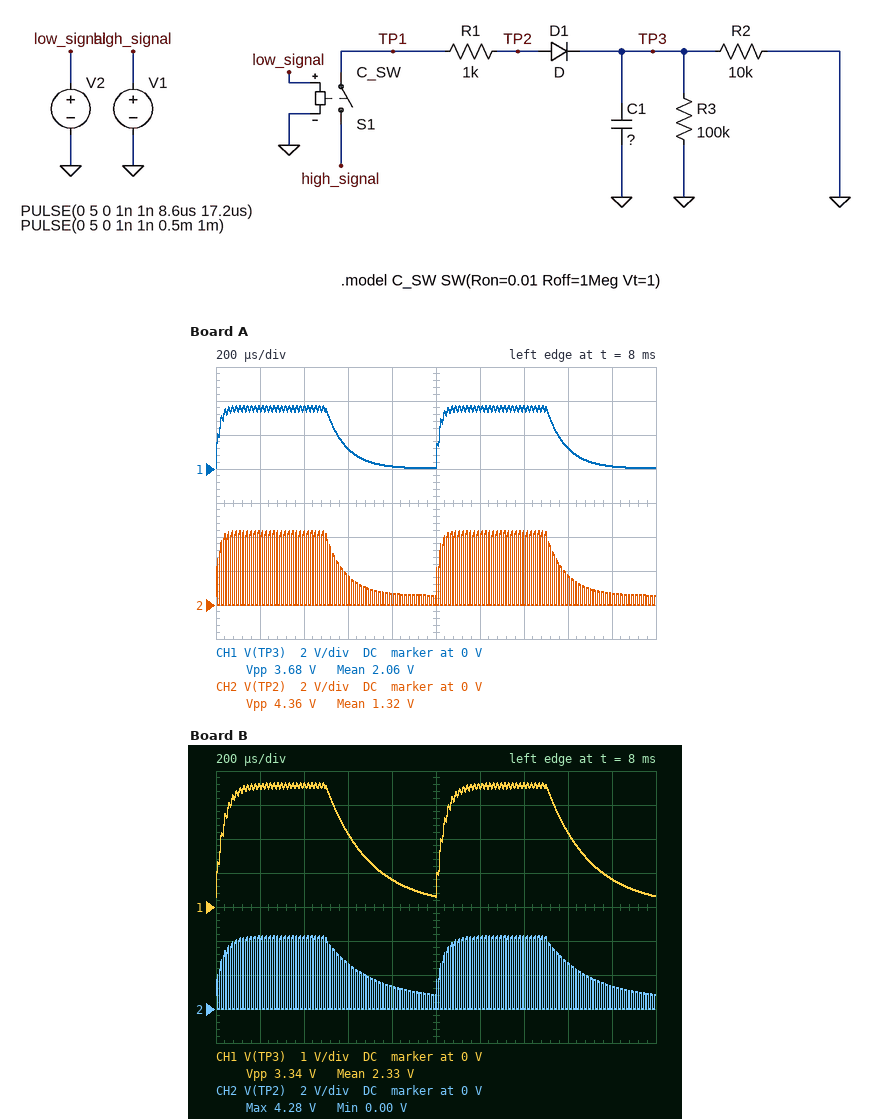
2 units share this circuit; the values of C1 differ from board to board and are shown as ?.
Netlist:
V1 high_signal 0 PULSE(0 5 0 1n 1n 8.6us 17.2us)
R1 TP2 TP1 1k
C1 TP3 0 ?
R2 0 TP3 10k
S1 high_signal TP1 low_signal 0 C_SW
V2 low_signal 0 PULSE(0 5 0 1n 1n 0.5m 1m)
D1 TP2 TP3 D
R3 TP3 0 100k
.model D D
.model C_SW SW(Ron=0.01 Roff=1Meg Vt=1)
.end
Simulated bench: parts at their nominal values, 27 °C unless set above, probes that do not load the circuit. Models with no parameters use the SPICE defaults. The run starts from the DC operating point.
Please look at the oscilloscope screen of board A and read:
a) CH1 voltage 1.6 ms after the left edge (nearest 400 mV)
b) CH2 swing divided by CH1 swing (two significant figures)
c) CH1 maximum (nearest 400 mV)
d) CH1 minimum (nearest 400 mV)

1.2 V
1.2
3.6 V
0 V
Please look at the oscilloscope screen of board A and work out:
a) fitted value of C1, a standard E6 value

10 nF
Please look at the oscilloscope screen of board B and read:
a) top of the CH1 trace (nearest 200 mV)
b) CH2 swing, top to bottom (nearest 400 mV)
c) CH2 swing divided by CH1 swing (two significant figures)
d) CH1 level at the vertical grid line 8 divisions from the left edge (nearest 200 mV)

3.6 V
4.4 V
1.3
2.2 V
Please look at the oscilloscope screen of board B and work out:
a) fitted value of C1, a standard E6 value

22 nF
